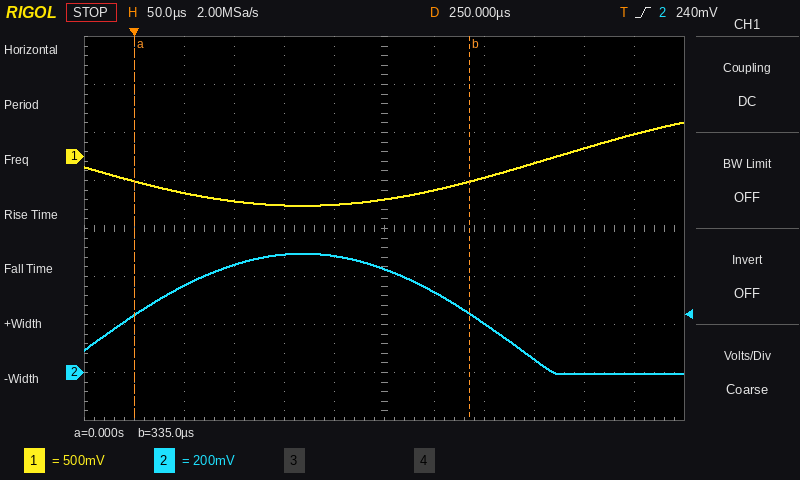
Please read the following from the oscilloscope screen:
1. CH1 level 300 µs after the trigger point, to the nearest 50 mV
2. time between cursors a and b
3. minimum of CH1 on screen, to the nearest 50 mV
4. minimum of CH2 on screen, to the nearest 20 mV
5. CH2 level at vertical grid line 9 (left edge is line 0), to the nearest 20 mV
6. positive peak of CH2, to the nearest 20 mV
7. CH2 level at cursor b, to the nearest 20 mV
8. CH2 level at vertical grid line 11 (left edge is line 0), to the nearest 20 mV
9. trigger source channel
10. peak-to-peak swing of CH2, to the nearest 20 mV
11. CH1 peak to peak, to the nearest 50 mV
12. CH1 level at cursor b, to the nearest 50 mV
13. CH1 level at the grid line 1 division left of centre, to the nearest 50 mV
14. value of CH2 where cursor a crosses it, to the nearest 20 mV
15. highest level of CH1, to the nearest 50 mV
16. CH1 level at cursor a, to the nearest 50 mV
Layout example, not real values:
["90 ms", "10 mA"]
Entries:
["-350 mV", "335 µs", "-500 mV", "0 mV", "60 mV", "500 mV", "240 mV", "0 mV", "CH2", "500 mV", "850 mV", "-250 mV", "-500 mV", "240 mV", "350 mV", "-250 mV"]
